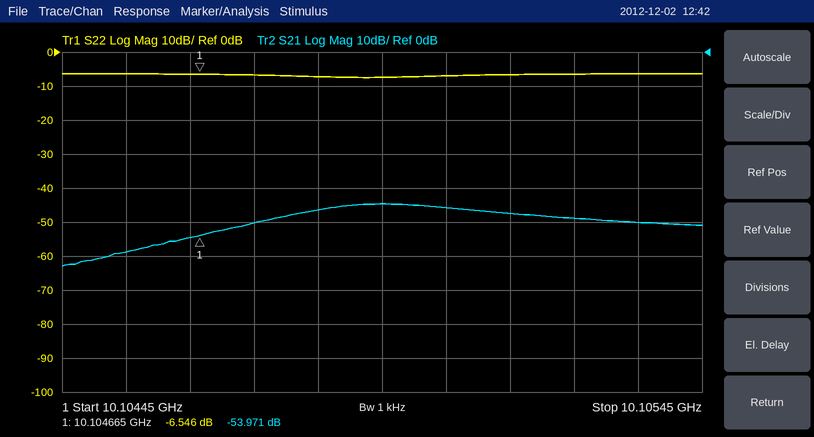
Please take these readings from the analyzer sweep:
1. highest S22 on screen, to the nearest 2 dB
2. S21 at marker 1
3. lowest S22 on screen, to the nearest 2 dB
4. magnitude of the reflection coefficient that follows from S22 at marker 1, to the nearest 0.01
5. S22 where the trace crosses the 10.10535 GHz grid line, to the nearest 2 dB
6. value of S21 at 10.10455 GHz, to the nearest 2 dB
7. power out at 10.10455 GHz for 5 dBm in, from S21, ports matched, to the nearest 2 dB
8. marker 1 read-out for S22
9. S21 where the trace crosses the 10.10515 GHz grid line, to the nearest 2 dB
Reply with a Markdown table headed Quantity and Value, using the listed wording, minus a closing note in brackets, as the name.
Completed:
| Quantity | Value |
|---|---|
| highest S22 on screen, to the nearest 2 dB | -6 dB |
| S21 at marker 1 | -53.971 dB |
| lowest S22 on screen, to the nearest 2 dB | -8 dB |
| magnitude of the reflection coefficient that follows from S22 at marker 1, to the nearest 0.01 | 0.47 |
| S22 where the trace crosses the 10.10535 GHz grid line, to the nearest 2 dB | -6 dB |
| value of S21 at 10.10455 GHz, to the nearest 2 dB | -58 dB |
| power out at 10.10455 GHz for 5 dBm in, from S21, ports matched, to the nearest 2 dB | -54 dBm |
| marker 1 read-out for S22 | -6.546 dB |
| S21 where the trace crosses the 10.10515 GHz grid line, to the nearest 2 dB | -48 dB |
